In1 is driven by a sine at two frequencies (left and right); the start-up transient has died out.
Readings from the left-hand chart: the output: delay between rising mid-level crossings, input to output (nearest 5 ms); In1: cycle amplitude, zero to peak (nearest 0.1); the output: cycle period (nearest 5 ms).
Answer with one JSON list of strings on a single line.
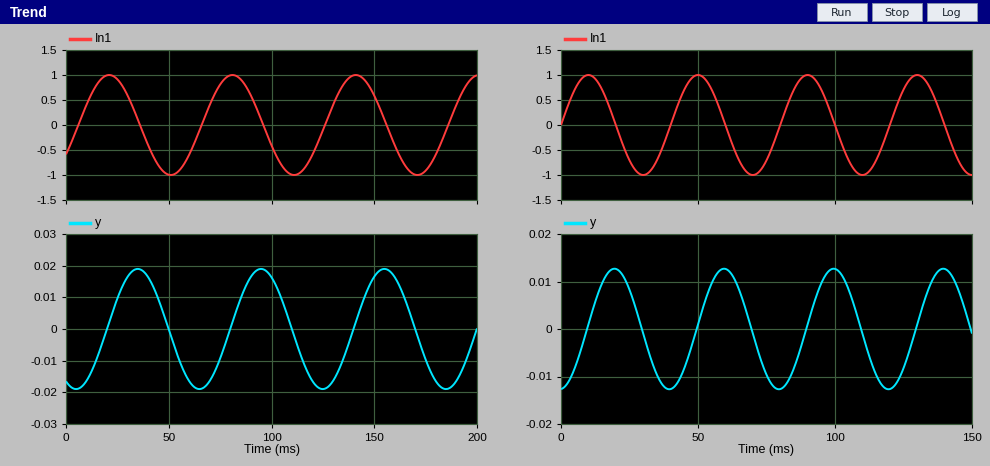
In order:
["15 ms", "1.0", "60 ms"]
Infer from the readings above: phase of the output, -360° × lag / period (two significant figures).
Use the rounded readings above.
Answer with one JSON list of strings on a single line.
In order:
["-90°"]
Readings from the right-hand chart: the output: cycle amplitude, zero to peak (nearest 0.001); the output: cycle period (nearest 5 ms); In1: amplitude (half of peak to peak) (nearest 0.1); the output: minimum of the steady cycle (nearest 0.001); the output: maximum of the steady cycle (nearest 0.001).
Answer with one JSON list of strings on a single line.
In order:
["0.013", "40 ms", "1.0", "-0.013", "0.013"]
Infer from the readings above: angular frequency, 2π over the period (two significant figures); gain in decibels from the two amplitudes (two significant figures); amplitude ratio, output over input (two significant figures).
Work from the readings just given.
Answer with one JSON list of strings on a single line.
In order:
["0.16 rad/ms", "-38 dB", "0.013"]
